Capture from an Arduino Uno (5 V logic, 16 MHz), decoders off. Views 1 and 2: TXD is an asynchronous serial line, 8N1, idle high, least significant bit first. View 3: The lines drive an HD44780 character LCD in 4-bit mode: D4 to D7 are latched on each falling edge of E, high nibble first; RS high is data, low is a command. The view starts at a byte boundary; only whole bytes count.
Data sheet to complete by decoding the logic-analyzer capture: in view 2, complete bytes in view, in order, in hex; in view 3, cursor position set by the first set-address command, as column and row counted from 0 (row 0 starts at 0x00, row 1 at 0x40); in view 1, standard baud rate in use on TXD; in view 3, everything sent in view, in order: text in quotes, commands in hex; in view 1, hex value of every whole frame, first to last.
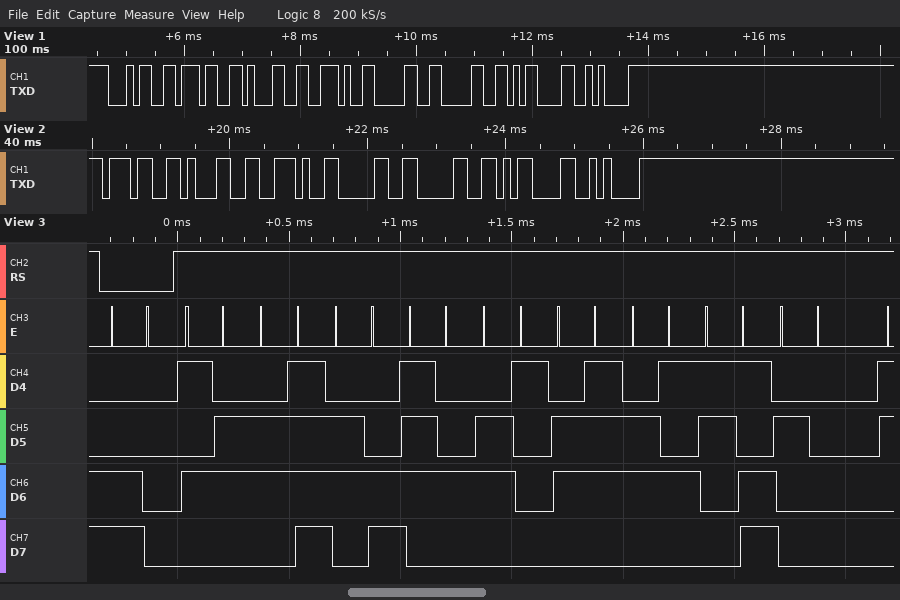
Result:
37 31 2E 30 30 0D 0A
column 0, row 1
9600 baud
0xC0 "Voltage= "
34 37 31 2E 30 30 0D 0A
